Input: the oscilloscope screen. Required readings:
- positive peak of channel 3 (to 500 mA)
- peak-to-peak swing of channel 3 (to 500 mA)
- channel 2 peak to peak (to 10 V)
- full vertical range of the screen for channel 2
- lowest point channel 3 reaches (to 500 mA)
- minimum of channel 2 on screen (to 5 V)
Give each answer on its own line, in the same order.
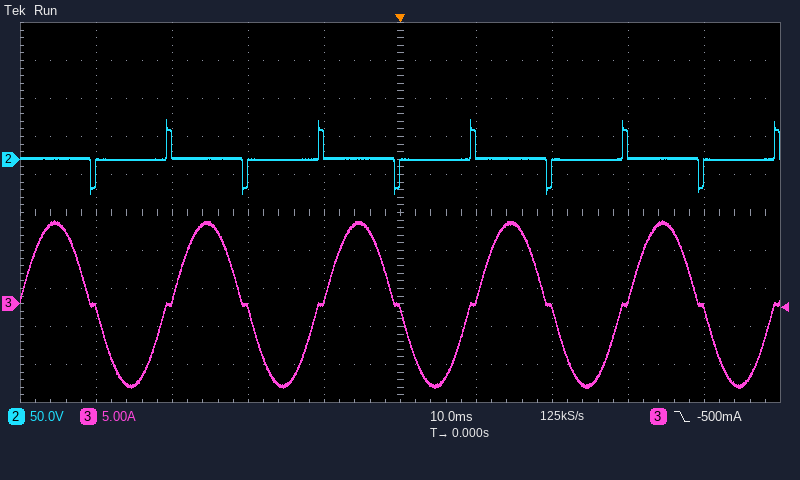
11.0 A
22.0 A
100 V
500 V
-11.0 A
-45 V
